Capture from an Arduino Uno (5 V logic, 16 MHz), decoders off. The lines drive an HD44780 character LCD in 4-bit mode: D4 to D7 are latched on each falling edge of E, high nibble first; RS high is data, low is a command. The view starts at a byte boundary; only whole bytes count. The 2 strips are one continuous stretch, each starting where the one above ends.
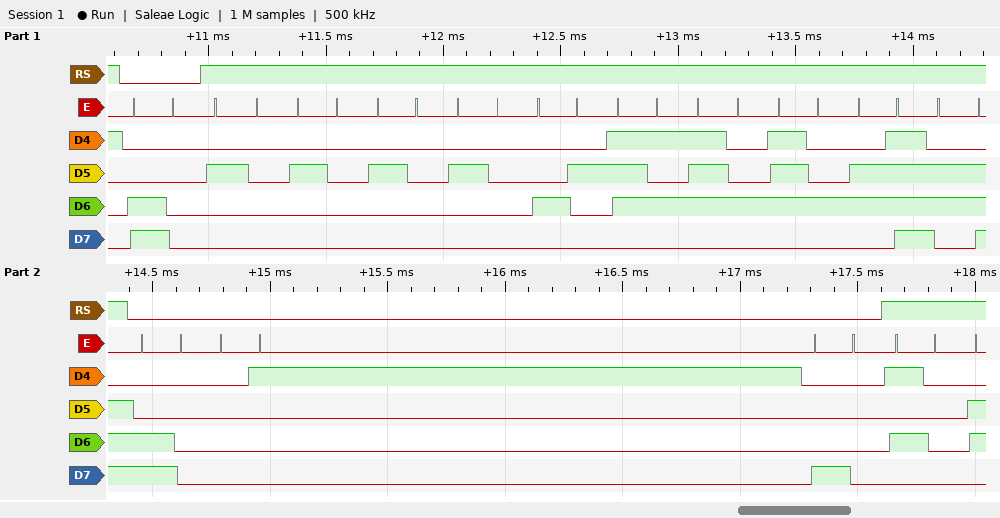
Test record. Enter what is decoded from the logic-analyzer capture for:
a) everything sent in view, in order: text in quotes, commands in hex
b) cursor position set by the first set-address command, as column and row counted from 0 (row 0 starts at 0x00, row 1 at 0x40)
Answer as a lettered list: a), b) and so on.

a) 0xC0 "    Button" 0xC0 0x01 0x80 "P"
b) column 0, row 1
